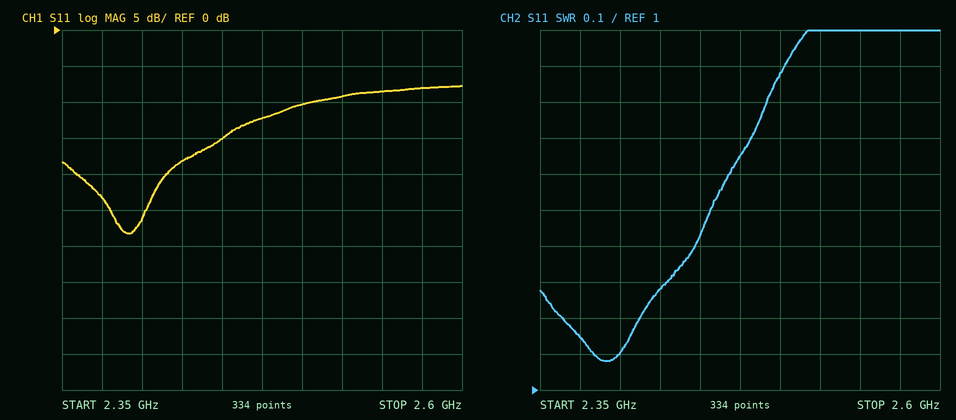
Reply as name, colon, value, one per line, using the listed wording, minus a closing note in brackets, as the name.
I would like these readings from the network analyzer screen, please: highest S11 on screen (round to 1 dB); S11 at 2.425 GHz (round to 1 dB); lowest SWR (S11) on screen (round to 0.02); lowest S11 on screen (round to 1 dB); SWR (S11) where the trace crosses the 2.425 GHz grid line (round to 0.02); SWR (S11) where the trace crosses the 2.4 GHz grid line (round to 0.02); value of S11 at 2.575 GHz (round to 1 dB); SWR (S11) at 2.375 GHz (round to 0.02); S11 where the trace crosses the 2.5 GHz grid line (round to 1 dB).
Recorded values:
highest S11 on screen: -8 dB
S11 at 2.425 GHz: -18 dB
lowest SWR (S11) on screen: 1.08
lowest S11 on screen: -28 dB
SWR (S11) where the trace crosses the 2.425 GHz grid line: 1.28
SWR (S11) where the trace crosses the 2.4 GHz grid line: 1.10
value of S11 at 2.575 GHz: -8 dB
SWR (S11) at 2.375 GHz: 1.14
S11 where the trace crosses the 2.5 GHz grid line: -10 dB
